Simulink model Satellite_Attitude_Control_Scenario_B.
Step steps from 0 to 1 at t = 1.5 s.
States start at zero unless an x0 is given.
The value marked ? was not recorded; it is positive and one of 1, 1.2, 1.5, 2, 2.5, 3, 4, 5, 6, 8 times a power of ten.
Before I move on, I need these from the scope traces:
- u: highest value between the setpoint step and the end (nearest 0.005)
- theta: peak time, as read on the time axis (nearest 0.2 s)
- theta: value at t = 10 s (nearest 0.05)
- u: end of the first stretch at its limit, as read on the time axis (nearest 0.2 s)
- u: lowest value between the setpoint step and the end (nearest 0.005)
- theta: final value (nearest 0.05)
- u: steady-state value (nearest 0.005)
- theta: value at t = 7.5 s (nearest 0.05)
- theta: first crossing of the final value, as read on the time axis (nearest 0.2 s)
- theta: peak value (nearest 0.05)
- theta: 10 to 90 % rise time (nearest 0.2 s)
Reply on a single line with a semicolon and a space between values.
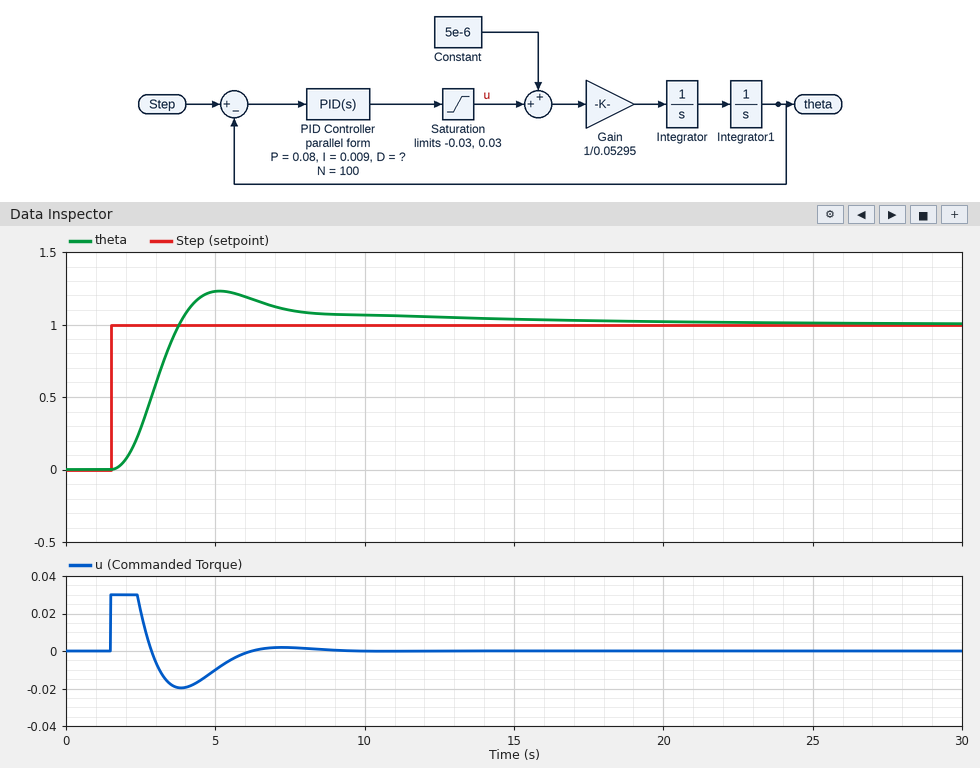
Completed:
0.030; 5.2 s; 1.05; 2.4 s; -0.020; 1.00; 0.000; 1.10; 3.8 s; 1.25; 1.4 s
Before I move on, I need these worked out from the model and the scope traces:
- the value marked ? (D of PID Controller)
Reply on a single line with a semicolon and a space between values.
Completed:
0.08
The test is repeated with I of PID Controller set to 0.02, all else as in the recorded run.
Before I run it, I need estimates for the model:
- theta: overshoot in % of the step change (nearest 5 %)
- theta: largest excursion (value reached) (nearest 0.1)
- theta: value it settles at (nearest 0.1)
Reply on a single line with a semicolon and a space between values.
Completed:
40 %; 1.4; 1.0
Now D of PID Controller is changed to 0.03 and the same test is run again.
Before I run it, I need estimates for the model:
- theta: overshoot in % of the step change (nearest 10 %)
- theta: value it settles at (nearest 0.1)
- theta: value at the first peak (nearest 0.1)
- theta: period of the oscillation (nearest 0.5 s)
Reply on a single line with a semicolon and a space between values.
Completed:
70 %; 1.0; 1.7; 5.5 s
